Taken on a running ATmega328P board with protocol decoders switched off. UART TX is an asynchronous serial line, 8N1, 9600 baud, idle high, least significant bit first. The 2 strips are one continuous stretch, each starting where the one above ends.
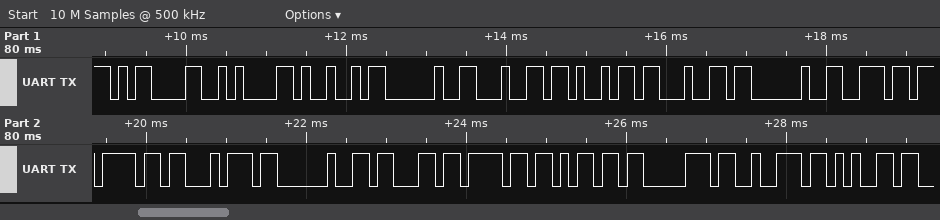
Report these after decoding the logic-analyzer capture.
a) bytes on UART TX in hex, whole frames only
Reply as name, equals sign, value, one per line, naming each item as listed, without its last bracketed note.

bytes on UART TX in hex, whole frames only = 0D 0A 49 20 64 69 64 20 6E 6F 74 20 63 6F 6D 70 72 65
